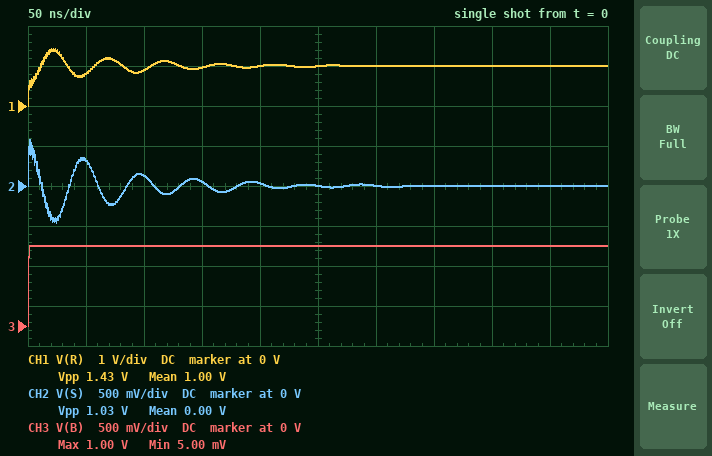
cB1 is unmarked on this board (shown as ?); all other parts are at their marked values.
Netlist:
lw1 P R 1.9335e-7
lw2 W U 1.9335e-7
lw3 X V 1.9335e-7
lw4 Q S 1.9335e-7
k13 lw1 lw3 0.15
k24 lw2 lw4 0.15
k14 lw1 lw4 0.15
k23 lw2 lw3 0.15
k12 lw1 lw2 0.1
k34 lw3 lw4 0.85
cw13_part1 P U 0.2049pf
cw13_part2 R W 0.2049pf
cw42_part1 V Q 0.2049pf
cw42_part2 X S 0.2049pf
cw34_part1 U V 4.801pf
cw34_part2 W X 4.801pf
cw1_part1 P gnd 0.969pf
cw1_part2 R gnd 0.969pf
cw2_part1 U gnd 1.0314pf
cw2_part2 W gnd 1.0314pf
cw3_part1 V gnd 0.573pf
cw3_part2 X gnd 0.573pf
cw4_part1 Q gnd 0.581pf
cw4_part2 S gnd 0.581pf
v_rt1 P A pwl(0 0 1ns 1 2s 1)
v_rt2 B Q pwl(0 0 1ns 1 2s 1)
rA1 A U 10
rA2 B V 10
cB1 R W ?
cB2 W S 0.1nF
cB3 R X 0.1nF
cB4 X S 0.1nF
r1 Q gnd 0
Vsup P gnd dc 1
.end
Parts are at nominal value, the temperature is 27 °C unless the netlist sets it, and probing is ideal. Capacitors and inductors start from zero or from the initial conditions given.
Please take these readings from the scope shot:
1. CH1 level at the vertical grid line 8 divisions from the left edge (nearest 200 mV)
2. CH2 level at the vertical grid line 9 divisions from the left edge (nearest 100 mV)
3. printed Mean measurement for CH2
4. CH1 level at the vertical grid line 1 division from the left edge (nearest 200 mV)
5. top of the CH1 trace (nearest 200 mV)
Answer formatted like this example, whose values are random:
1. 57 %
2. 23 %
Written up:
1. 1.0 V
2. 0 V
3. 0.00 V
4. 800 mV
5. 1.4 V
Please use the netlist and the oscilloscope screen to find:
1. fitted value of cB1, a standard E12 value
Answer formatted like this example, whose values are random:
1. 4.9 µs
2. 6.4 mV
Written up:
1. 180 pF
